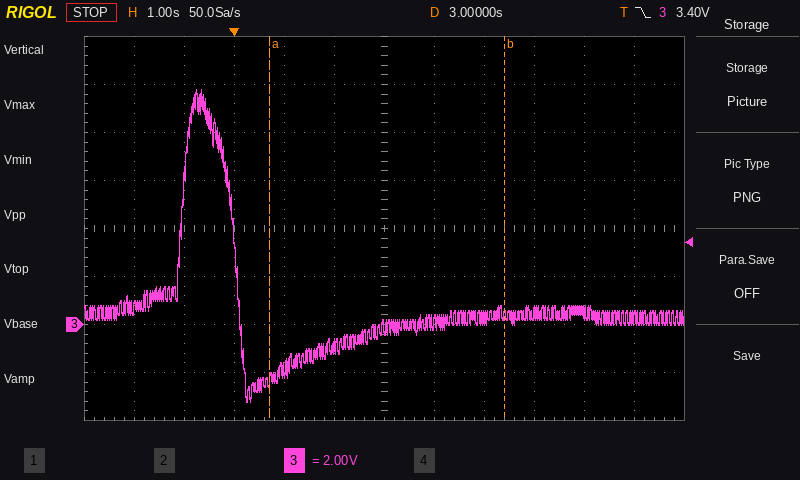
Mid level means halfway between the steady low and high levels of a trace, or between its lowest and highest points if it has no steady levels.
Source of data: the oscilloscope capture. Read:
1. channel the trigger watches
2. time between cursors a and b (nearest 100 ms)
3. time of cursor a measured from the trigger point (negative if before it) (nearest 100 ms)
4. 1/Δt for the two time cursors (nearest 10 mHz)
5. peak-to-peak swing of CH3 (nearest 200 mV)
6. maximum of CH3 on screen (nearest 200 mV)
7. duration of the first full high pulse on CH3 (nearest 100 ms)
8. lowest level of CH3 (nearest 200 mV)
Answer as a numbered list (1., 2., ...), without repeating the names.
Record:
1. CH3
2. 4.7 s
3. +700 ms
4. 210 mHz
5. 13.0 V
6. 9.8 V
7. 1.1 s
8. -3.2 V
